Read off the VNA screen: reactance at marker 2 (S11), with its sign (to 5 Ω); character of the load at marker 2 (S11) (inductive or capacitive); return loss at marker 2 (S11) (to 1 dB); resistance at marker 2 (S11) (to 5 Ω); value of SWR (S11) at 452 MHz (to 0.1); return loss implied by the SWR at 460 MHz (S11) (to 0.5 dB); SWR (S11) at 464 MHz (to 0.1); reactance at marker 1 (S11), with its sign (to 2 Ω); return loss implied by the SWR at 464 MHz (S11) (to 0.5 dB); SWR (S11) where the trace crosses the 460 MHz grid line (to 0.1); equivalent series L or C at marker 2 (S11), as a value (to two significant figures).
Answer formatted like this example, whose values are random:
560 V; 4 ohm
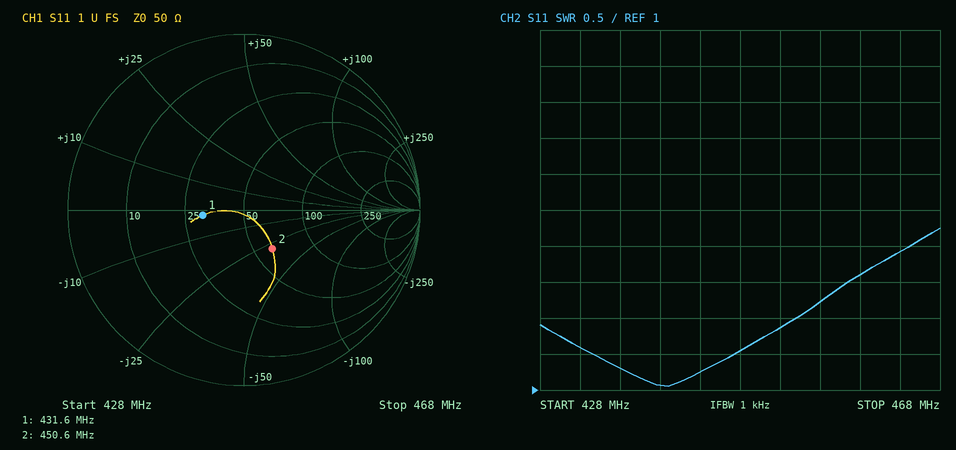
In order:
-30 Ω; capacitive; 11 dB; 60 Ω; 1.9; 7.0 dB; 2.9; -2 Ω; 6.0 dB; 2.6; 12 pF
